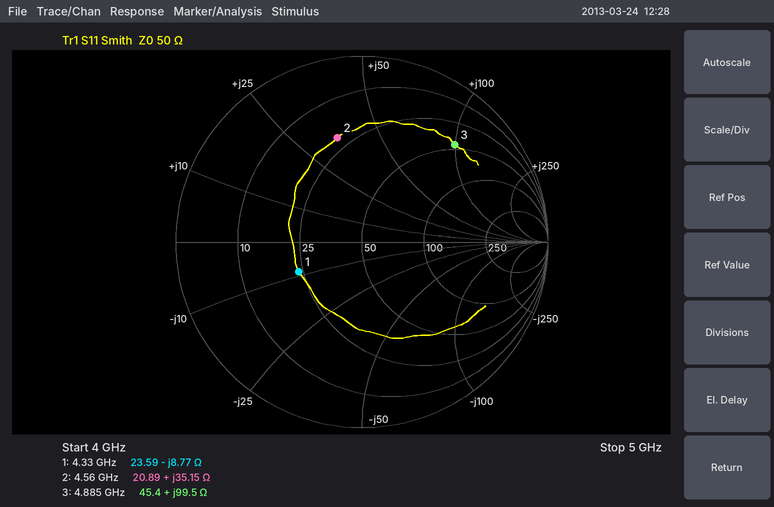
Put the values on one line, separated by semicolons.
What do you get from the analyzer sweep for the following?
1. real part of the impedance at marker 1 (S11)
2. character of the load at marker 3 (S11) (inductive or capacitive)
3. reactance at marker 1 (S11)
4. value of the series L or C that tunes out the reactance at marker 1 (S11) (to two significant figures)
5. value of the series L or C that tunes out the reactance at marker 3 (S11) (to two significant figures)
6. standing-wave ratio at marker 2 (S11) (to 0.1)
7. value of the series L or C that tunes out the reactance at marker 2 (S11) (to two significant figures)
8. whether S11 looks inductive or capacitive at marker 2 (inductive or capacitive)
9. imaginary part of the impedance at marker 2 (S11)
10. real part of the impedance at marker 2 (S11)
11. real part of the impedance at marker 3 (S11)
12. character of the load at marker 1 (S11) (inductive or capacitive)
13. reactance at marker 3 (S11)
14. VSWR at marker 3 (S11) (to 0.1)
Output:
23.59 Ω; inductive; -8.77 Ω; 320 pH; 330 fF; 3.7; 990 fF; inductive; +35.15 Ω; 20.89 Ω; 45.4 Ω; capacitive; +99.5 Ω; 6.2
